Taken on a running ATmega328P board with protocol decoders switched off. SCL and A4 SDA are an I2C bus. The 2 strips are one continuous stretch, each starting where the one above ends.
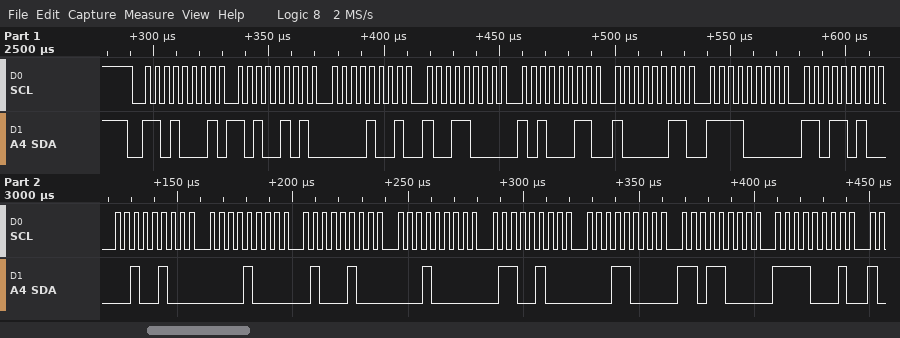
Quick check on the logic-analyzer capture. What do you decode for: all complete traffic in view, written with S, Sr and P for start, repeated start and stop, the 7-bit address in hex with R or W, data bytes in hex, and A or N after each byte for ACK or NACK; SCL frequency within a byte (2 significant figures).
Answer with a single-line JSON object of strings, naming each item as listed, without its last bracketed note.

{"all complete traffic in view, written with S, Sr and P for start, repeated start and stop, the 7-bit address in hex with R or W, data bytes in hex, and A or N after each byte for ACK or NACK": "S 68R A A5 A 09 A 98 A A3 A 83 A F0 A DA A 24 A 08 A 44 A 10 A 64 A 18 A D8 A F1 A", "SCL frequency within a byte": "250 kHz"}
